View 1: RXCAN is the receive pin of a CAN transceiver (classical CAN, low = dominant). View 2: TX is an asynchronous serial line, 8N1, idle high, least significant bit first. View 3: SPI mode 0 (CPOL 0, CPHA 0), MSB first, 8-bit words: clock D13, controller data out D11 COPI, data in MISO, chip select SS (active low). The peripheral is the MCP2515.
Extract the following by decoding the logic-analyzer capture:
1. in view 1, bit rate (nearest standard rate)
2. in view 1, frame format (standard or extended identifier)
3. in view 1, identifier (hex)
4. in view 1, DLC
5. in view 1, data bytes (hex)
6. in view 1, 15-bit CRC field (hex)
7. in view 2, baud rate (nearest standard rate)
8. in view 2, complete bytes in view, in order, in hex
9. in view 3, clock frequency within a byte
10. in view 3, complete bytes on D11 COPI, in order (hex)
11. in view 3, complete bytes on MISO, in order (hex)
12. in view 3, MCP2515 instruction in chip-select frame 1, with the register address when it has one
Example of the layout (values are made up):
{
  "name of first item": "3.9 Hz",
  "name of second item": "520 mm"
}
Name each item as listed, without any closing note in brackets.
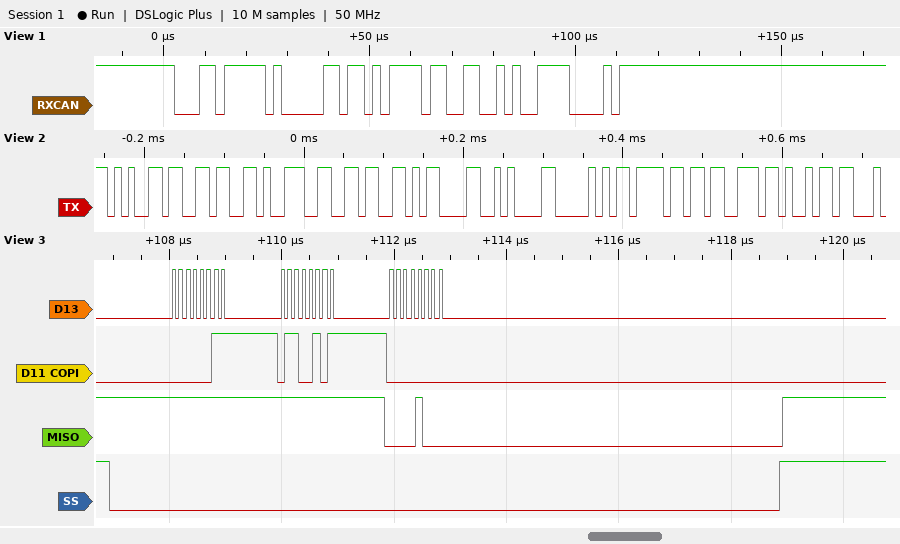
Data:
{
  "in view 1, bit rate": "500 kbit/s",
  "in view 1, frame format": "standard",
  "in view 1, identifier": "0x1BF",
  "in view 1, DLC": "2",
  "in view 1, data bytes": "D7 B3",
  "in view 1, 15-bit CRC field": "0x14F0",
  "in view 2, baud rate": "115200 baud",
  "in view 2, complete bytes in view, in order, in hex": "65 36 39 36 0D 0A 50 6F 73 69",
  "in view 3, clock frequency within a byte": "8 MHz",
  "in view 3, complete bytes on D11 COPI, in order": "03 65 00",
  "in view 3, complete bytes on MISO, in order": "FF FF 08",
  "in view 3, MCP2515 instruction in chip-select frame 1, with the register address when it has one": "READ 0x65"
}
